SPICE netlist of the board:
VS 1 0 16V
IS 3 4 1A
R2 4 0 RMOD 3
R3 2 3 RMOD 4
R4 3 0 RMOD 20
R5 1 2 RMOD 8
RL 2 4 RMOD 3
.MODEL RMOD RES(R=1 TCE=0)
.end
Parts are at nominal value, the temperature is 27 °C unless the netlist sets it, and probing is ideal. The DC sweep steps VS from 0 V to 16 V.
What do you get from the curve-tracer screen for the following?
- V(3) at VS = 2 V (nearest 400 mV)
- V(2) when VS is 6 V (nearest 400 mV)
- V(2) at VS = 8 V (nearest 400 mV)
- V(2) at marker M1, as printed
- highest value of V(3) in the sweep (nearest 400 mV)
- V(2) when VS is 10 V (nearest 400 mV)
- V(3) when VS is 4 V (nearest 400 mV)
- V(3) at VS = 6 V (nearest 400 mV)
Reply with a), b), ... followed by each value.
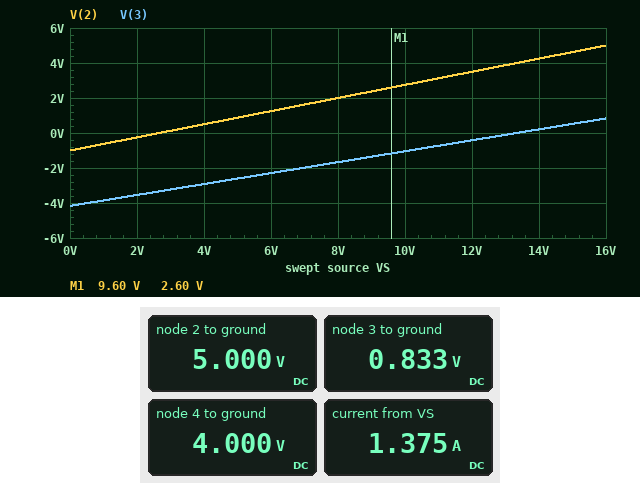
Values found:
a) -3.6 V
b) 1.2 V
c) 2.0 V
d) 2.60 V
e) 800 mV
f) 2.8 V
g) -2.8 V
h) -2.4 V
